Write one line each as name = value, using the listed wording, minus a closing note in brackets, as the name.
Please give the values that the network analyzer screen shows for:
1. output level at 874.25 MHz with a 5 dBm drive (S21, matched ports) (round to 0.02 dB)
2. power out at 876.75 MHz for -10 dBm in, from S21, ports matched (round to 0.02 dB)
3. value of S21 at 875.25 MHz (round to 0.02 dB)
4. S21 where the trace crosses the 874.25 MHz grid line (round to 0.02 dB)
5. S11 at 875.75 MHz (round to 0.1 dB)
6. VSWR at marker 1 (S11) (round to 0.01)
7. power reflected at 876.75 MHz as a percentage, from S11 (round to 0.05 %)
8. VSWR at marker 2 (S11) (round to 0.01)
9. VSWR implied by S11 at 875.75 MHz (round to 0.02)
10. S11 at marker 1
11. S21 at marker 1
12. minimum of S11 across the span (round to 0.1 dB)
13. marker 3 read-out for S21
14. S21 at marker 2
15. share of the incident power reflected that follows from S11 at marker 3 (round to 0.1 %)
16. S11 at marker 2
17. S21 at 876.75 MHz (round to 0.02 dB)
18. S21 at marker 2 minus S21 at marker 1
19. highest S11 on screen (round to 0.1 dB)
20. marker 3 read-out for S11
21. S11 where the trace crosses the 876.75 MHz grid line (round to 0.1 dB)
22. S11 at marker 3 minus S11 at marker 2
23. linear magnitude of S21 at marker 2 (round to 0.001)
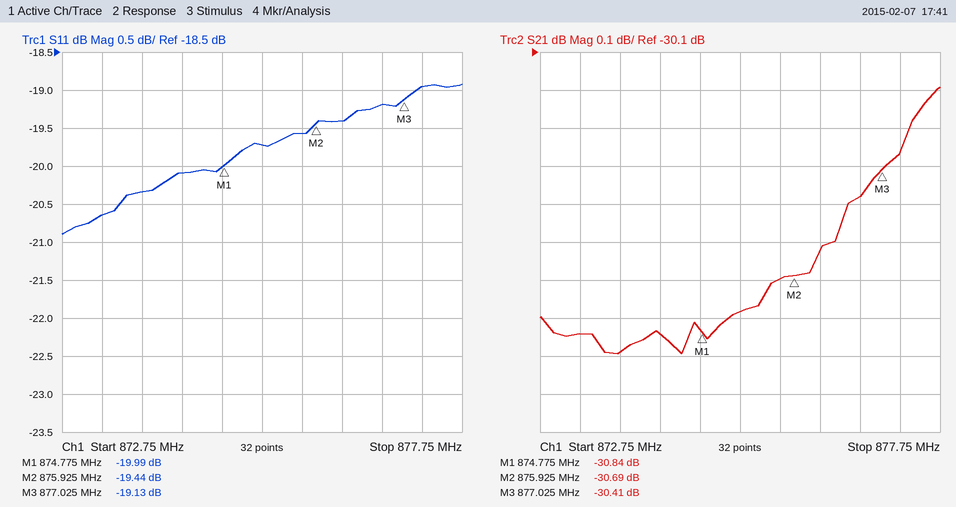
output level at 874.25 MHz with a 5 dBm drive (S21, matched ports) = -25.84 dBm
power out at 876.75 MHz for -10 dBm in, from S21, ports matched = -40.48 dBm
value of S21 at 875.25 MHz = -30.78 dB
S21 where the trace crosses the 874.25 MHz grid line = -30.84 dB
S11 at 875.75 MHz = -19.6 dB
VSWR at marker 1 (S11) = 1.22
power reflected at 876.75 MHz as a percentage, from S11 = 1.20 %
VSWR at marker 2 (S11) = 1.24
VSWR implied by S11 at 875.75 MHz = 1.24
S11 at marker 1 = -19.99 dB
S21 at marker 1 = -30.84 dB
minimum of S11 across the span = -20.9 dB
marker 3 read-out for S21 = -30.41 dB
S21 at marker 2 = -30.69 dB
share of the incident power reflected that follows from S11 at marker 3 = 1.2 %
S11 at marker 2 = -19.44 dB
S21 at 876.75 MHz = -30.48 dB
S21 at marker 2 minus S21 at marker 1 = 0.15 dB
highest S11 on screen = -18.9 dB
marker 3 read-out for S11 = -19.13 dB
S11 where the trace crosses the 876.75 MHz grid line = -19.2 dB
S11 at marker 3 minus S11 at marker 2 = 0.31 dB
linear magnitude of S21 at marker 2 = 0.029
